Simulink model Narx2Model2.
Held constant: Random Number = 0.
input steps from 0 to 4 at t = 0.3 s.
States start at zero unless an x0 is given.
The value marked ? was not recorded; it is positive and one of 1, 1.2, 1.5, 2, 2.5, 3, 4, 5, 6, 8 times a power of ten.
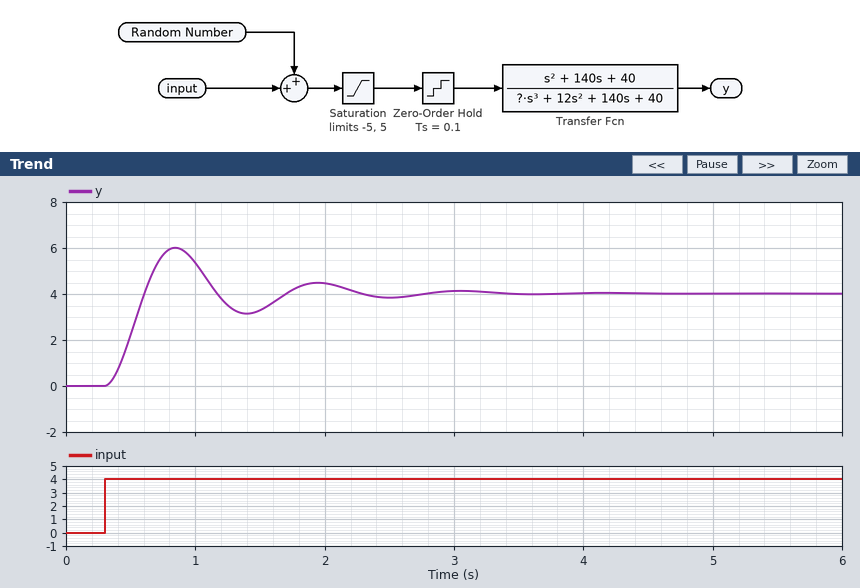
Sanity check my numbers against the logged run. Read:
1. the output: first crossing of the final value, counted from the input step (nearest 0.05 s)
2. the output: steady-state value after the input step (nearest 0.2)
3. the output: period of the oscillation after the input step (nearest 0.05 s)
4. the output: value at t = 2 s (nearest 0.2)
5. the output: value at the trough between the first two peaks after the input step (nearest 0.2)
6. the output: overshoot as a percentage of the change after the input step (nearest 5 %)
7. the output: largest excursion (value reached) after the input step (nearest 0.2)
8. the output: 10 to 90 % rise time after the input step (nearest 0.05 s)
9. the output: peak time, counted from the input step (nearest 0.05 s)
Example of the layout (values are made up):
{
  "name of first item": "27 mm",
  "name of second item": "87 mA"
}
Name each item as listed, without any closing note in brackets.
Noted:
{
  "the output: first crossing of the final value, counted from the input step": "0.30 s",
  "the output: steady-state value after the input step": "4.0",
  "the output: period of the oscillation after the input step": "1.10 s",
  "the output: value at t = 2 s": "4.4",
  "the output: value at the trough between the first two peaks after the input step": "3.2",
  "the output: overshoot as a percentage of the change after the input step": "50 %",
  "the output: largest excursion (value reached) after the input step": "6.0",
  "the output: 10 to 90 % rise time after the input step": "0.20 s",
  "the output: peak time, counted from the input step": "0.55 s"
}
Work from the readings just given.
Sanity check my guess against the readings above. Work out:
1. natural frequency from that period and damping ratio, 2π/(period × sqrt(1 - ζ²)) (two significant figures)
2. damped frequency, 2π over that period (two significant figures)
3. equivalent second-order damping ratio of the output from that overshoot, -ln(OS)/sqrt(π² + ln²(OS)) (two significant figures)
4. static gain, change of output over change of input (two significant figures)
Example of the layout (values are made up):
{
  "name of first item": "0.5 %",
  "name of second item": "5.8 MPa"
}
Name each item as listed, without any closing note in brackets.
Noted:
{
  "natural frequency from that period and damping ratio, 2π/(period × sqrt(1 - ζ²))": "5.9 rad/s",
  "damped frequency, 2π over that period": "5.7 rad/s",
  "equivalent second-order damping ratio of the output from that overshoot, -ln(OS)/sqrt(π² + ln²(OS))": "0.22",
  "static gain, change of output over change of input": "1.0"
}
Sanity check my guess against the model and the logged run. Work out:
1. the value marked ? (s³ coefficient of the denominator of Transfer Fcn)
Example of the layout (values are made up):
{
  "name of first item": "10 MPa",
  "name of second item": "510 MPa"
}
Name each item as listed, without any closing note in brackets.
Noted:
{
  "the value marked ?": "4"
}
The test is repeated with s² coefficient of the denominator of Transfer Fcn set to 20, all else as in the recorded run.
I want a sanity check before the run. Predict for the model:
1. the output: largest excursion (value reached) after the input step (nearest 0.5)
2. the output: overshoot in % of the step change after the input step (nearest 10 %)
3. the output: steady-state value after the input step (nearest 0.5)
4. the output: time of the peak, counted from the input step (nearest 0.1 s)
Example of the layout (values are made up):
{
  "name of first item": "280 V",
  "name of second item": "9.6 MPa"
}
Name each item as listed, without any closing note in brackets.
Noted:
{
  "the output: largest excursion (value reached) after the input step": "5.0",
  "the output: overshoot in % of the step change after the input step": "30 %",
  "the output: steady-state value after the input step": "4.0",
  "the output: time of the peak, counted from the input step": "0.6 s"
}
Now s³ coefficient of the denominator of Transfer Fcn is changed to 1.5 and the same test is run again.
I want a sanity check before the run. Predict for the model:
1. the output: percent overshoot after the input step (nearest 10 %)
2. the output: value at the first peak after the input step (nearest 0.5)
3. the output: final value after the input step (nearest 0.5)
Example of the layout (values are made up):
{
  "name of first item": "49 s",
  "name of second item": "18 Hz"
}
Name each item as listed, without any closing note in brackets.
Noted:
{
  "the output: percent overshoot after the input step": "30 %",
  "the output: value at the first peak after the input step": "5.0",
  "the output: final value after the input step": "4.0"
}
